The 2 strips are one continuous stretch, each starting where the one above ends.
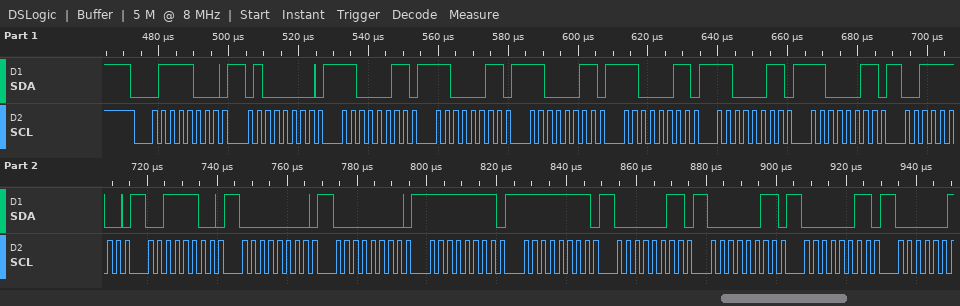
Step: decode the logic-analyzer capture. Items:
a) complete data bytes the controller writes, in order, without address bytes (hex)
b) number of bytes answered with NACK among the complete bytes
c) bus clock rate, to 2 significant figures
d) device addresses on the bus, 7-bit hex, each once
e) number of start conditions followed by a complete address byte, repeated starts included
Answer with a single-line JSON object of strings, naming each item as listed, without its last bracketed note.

{"complete data bytes the controller writes, in order, without address bytes": "40 C3 C3 C3 C3 C3 C3 3C 3C 00 00 FF FF 03 03 03", "number of bytes answered with NACK among the complete bytes": "0", "bus clock rate, to 2 significant figures": "400 kHz", "device addresses on the bus, 7-bit hex, each once": "0x3C", "number of start conditions followed by a complete address byte, repeated starts included": "1"}
